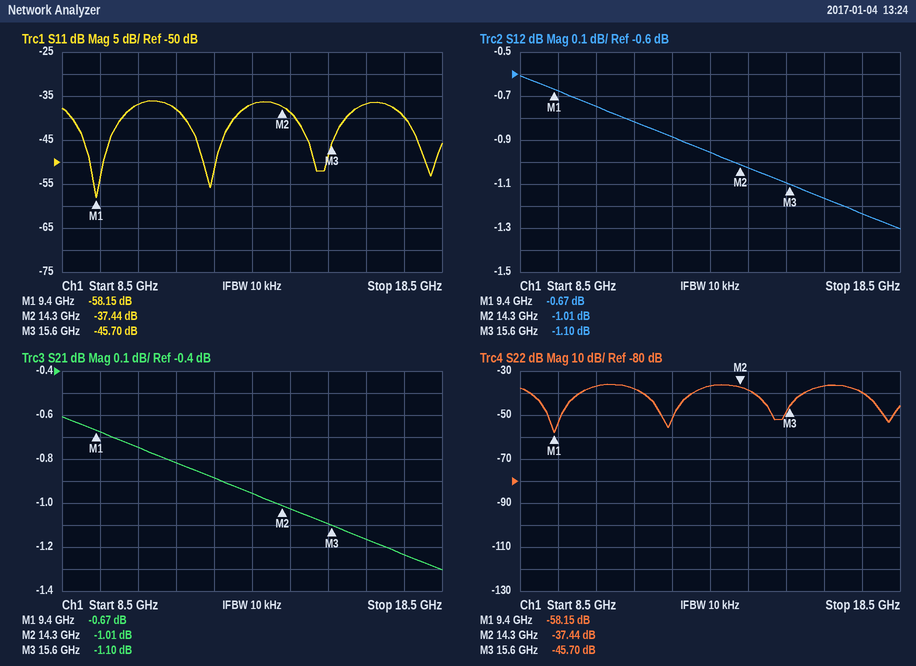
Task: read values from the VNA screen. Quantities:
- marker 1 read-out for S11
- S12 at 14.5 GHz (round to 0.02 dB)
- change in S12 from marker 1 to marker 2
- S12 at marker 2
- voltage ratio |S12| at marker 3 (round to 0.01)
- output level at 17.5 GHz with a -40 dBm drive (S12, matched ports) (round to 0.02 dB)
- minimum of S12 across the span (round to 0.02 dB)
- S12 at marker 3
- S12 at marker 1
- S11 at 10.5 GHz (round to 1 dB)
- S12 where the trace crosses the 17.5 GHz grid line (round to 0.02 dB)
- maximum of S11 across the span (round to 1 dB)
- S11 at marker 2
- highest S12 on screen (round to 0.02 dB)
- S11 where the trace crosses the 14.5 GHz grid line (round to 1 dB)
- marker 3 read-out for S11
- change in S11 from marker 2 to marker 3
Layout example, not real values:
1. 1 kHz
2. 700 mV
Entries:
1. -58.15 dB
2. -1.02 dB
3. -0.34 dB
4. -1.01 dB
5. 0.88
6. -41.24 dBm
7. -1.30 dB
8. -1.10 dB
9. -0.67 dB
10. -37 dB
11. -1.24 dB
12. -36 dB
13. -37.44 dB
14. -0.60 dB
15. -39 dB
16. -45.70 dB
17. -8.26 dB
